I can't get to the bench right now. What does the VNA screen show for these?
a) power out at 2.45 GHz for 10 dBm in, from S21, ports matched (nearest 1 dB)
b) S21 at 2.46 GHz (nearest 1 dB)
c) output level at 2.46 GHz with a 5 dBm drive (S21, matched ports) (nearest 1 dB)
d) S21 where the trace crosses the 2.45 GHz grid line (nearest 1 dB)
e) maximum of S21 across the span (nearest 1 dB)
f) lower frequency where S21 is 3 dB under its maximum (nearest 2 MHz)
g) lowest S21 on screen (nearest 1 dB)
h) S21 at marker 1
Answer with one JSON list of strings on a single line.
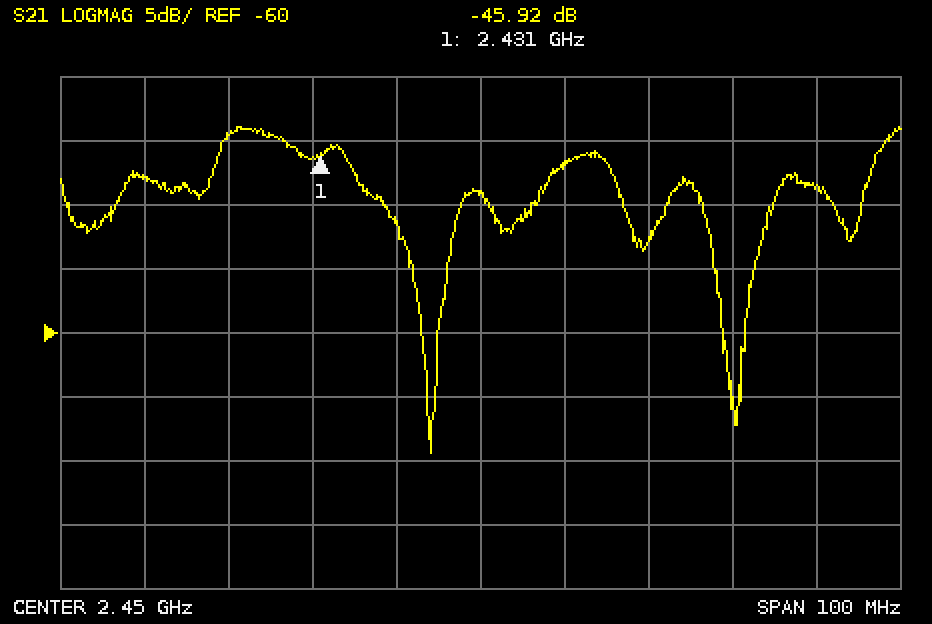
["-39 dBm", "-47 dB", "-42 dBm", "-49 dB", "-44 dB", "2.418 GHz", "-69 dB", "-45.92 dB"]
